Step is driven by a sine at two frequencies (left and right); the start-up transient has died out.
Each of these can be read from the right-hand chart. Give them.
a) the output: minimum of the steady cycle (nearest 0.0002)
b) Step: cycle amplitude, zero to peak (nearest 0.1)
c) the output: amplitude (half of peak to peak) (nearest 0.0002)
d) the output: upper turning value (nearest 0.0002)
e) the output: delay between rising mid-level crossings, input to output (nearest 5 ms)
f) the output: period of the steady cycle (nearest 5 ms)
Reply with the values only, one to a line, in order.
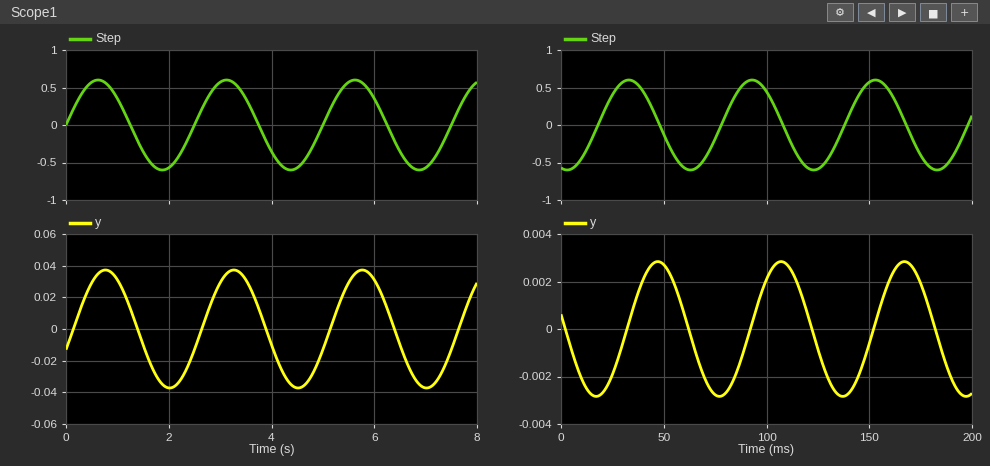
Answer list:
-0.0028
0.6
0.0028
0.0028
15 ms
60 ms
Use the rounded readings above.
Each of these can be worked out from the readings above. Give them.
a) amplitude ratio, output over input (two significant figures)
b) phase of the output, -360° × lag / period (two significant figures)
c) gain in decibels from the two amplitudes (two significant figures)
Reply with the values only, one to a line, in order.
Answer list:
0.0047
-90°
-47 dB
